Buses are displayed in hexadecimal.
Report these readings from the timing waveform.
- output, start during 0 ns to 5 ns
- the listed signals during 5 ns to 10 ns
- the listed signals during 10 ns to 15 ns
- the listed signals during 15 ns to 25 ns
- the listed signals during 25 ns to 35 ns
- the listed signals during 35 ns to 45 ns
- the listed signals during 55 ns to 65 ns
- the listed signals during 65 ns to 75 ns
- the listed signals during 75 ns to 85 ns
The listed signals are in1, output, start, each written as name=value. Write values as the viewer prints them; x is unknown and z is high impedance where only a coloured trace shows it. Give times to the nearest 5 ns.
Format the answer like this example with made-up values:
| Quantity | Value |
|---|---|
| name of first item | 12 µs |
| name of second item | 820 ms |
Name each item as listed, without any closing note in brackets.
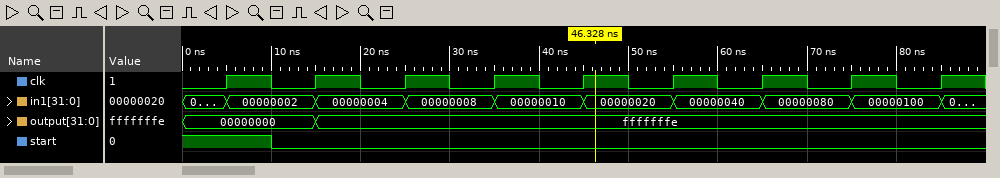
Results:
| Quantity | Value |
|---|---|
| output, start during 0 ns to 5 ns | output=00000000, start=1 |
| the listed signals during 5 ns to 10 ns | in1=00000002, output=00000000, start=1 |
| the listed signals during 10 ns to 15 ns | in1=00000002, output=00000000, start=0 |
| the listed signals during 15 ns to 25 ns | in1=00000004, output=fffffffe, start=0 |
| the listed signals during 25 ns to 35 ns | in1=00000008, output=fffffffe, start=0 |
| the listed signals during 35 ns to 45 ns | in1=00000010, output=fffffffe, start=0 |
| the listed signals during 55 ns to 65 ns | in1=00000040, output=fffffffe, start=0 |
| the listed signals during 65 ns to 75 ns | in1=00000080, output=fffffffe, start=0 |
| the listed signals during 75 ns to 85 ns | in1=00000100, output=fffffffe, start=0 |
